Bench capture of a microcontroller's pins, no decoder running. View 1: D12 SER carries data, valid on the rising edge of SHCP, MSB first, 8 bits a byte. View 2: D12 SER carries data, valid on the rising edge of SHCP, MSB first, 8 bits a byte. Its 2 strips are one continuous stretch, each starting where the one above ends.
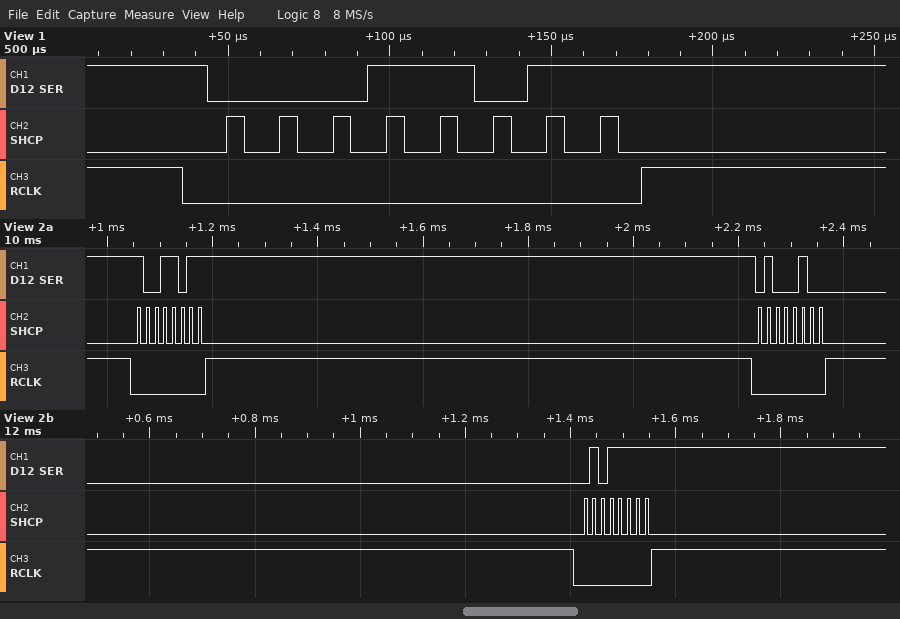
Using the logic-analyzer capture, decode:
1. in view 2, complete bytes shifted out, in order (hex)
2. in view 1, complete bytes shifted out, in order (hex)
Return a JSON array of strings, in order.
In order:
["9B 44 5F", "1B"]
